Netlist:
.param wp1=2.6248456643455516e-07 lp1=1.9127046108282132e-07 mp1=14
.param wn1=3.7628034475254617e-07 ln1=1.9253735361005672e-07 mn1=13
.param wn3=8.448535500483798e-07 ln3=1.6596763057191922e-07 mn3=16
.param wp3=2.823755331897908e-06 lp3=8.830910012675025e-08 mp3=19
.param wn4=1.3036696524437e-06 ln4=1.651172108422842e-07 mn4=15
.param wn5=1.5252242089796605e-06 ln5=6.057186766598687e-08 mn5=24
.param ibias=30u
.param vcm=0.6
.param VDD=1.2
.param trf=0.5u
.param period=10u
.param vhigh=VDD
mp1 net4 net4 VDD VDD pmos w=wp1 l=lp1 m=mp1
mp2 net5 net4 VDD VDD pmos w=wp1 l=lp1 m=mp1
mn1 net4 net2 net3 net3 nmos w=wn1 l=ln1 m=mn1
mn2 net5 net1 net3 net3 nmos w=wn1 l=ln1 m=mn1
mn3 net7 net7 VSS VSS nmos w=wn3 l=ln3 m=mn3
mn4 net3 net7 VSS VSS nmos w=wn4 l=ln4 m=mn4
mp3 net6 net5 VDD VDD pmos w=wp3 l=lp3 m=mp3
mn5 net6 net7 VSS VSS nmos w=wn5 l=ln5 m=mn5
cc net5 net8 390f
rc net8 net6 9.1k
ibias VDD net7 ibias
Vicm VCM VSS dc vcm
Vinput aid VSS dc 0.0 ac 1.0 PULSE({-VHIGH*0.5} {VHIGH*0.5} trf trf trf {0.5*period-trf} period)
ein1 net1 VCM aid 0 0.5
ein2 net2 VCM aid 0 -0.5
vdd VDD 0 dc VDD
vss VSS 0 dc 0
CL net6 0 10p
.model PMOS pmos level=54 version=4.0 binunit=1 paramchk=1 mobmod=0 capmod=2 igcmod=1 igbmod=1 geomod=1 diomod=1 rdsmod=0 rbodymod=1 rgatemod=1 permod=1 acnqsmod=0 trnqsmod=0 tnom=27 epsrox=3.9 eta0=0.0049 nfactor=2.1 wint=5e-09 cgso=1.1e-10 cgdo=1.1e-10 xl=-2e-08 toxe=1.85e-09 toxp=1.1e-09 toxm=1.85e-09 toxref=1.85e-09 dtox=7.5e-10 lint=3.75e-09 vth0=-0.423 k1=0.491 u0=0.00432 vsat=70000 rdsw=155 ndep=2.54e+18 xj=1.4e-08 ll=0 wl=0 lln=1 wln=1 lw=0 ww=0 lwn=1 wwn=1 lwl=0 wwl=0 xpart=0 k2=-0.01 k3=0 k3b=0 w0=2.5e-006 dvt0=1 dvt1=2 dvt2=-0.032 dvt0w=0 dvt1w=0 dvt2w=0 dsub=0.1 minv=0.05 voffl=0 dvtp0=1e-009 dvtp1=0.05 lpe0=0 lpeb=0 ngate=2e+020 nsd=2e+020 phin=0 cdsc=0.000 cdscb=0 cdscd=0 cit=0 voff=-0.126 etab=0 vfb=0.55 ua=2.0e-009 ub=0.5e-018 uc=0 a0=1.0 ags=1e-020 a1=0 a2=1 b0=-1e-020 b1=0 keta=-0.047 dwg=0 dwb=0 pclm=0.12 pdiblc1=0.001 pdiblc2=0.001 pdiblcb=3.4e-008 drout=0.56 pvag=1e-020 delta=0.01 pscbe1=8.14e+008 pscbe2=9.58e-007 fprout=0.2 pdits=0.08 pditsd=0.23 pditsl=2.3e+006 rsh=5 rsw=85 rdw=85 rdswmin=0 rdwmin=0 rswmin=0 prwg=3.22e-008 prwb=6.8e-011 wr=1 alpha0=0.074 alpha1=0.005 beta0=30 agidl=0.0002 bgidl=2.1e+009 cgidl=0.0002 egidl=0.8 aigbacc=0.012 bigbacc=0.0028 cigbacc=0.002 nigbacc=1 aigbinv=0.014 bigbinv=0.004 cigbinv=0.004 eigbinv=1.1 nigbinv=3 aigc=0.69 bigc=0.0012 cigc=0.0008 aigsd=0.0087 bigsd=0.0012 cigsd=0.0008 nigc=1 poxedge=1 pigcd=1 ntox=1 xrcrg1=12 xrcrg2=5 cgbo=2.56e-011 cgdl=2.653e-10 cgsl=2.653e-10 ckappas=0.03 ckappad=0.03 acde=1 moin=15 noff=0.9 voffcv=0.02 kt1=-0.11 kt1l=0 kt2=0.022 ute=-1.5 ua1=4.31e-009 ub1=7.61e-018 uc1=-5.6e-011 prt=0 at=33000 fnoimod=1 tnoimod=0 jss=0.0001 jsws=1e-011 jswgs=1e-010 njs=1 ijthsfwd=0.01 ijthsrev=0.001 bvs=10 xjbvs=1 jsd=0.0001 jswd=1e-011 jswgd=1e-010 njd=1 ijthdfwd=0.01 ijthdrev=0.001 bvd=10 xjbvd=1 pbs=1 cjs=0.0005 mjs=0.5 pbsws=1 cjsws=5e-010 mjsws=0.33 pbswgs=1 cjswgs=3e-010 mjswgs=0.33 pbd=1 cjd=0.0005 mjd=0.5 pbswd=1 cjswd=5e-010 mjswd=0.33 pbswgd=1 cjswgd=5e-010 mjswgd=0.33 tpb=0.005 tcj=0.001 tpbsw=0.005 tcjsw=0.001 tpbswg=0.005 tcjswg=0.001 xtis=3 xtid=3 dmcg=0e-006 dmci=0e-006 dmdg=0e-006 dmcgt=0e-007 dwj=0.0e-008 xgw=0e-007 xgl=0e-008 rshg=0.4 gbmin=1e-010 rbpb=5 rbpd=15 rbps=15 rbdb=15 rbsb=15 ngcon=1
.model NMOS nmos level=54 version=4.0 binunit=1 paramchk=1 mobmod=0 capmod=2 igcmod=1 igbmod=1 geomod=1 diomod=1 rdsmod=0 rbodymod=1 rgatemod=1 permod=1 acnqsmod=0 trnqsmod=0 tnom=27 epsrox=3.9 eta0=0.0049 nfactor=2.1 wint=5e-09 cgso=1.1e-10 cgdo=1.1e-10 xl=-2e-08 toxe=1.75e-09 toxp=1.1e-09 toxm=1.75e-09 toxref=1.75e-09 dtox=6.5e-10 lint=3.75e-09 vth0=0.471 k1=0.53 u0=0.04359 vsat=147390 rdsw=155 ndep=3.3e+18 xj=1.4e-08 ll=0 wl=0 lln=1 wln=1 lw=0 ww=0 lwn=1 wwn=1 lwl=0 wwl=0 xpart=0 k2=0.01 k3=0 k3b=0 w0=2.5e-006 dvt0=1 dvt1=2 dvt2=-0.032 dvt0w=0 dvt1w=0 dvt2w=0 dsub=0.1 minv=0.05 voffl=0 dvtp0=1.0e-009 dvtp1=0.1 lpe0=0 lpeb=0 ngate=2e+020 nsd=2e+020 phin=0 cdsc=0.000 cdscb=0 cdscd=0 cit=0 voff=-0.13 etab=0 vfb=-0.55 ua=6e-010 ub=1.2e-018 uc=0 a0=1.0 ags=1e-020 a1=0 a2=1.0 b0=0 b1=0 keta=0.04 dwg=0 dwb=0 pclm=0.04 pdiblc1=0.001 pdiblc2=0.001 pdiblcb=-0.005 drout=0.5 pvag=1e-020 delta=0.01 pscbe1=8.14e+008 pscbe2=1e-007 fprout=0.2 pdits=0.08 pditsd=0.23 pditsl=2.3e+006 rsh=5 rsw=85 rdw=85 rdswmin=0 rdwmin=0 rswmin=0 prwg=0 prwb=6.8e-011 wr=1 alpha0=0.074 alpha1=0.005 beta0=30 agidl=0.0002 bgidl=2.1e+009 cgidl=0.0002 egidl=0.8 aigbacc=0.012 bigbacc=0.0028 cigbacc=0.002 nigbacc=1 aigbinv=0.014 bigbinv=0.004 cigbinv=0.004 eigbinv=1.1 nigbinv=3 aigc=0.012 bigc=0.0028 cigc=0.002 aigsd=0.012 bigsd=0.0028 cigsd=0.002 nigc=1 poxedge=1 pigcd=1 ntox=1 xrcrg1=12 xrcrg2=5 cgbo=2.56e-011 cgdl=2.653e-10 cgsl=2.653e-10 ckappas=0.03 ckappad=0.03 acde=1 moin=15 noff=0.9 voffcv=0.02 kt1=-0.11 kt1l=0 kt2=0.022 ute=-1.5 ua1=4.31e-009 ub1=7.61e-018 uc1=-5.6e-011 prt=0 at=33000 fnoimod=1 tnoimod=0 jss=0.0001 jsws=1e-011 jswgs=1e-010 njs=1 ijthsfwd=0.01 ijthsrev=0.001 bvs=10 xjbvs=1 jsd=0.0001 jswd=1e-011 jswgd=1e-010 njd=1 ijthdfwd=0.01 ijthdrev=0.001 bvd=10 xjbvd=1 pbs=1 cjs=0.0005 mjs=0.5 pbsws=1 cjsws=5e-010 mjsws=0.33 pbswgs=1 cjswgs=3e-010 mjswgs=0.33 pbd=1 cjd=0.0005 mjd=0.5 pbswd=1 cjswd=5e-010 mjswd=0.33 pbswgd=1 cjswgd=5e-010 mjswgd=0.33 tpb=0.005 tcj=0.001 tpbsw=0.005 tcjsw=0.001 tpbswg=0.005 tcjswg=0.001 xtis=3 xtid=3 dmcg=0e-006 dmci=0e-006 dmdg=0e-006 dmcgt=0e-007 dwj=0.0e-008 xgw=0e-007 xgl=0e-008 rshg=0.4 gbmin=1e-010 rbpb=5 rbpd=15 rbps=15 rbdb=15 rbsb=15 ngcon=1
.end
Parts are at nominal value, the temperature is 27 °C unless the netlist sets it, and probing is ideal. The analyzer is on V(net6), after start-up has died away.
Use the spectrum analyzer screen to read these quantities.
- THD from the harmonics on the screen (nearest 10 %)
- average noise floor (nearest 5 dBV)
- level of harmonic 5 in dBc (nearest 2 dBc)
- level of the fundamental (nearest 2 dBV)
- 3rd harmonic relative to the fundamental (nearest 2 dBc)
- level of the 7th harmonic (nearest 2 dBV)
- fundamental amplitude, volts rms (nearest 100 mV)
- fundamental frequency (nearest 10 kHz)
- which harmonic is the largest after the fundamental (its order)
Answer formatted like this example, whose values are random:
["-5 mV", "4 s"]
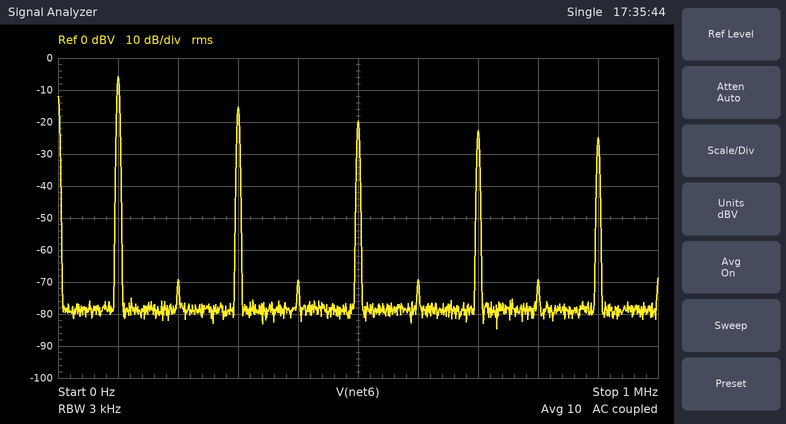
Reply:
["40 %", "-80 dBV", "-14 dBc", "-6 dBV", "-10 dBc", "-22 dBV", "500 mV", "100 kHz", "3"]
